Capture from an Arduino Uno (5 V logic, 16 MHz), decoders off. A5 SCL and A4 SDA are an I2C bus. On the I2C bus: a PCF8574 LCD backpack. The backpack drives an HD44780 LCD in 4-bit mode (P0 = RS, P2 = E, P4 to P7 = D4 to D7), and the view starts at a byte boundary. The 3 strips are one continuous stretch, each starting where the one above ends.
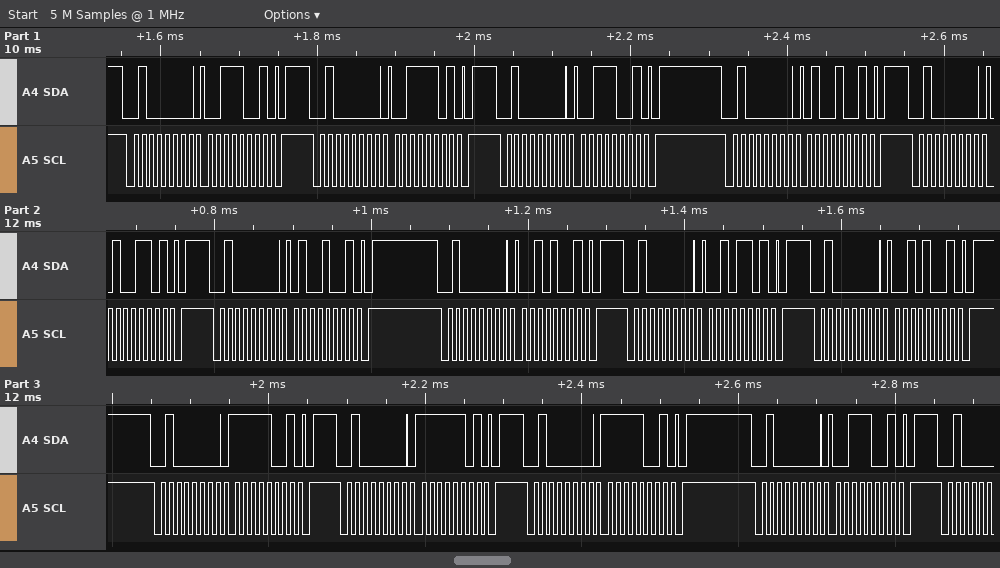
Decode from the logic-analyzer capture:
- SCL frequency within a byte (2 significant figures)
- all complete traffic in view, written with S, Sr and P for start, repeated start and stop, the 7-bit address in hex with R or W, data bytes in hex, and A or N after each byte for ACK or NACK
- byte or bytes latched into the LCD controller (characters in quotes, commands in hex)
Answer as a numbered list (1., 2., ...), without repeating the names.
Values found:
1. 100 kHz
2. S 20W A 39 A P S 20W A 3D A P S 20W A 39 A P S 20W A 49 A P S 20W A 4D A P S 20W A 49 A P S 20W A 29 A P S 20W A 2D A P S 20W A 29 A P S 20W A F9 A P S 20W A FD A P S 20W A F9 A P S 20W A 39 A P
3. '4' '/'
